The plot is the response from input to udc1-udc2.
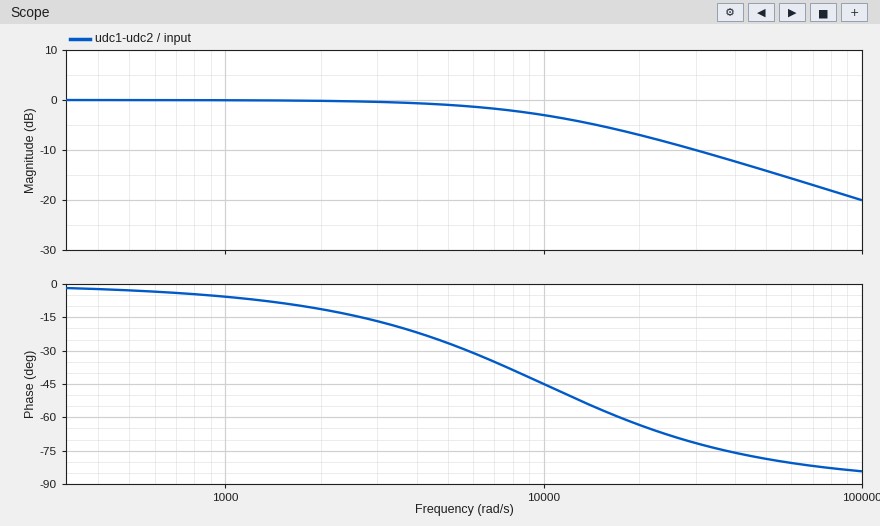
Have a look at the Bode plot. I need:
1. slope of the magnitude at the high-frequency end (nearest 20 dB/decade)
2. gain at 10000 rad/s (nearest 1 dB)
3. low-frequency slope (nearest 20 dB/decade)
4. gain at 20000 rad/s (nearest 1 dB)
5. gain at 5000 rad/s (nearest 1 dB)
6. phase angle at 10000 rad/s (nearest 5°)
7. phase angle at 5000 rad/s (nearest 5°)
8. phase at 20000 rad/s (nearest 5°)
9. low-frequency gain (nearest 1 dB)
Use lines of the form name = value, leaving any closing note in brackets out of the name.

slope of the magnitude at the high-frequency end = -20 dB/decade
gain at 10000 rad/s = -3 dB
low-frequency slope = 0 dB/decade
gain at 20000 rad/s = -7 dB
gain at 5000 rad/s = -1 dB
phase angle at 10000 rad/s = -45°
phase angle at 5000 rad/s = -25°
phase at 20000 rad/s = -65°
low-frequency gain = 0 dB
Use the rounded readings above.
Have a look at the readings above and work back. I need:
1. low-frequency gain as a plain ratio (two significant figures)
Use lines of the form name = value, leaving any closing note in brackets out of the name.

low-frequency gain as a plain ratio = 1.0
